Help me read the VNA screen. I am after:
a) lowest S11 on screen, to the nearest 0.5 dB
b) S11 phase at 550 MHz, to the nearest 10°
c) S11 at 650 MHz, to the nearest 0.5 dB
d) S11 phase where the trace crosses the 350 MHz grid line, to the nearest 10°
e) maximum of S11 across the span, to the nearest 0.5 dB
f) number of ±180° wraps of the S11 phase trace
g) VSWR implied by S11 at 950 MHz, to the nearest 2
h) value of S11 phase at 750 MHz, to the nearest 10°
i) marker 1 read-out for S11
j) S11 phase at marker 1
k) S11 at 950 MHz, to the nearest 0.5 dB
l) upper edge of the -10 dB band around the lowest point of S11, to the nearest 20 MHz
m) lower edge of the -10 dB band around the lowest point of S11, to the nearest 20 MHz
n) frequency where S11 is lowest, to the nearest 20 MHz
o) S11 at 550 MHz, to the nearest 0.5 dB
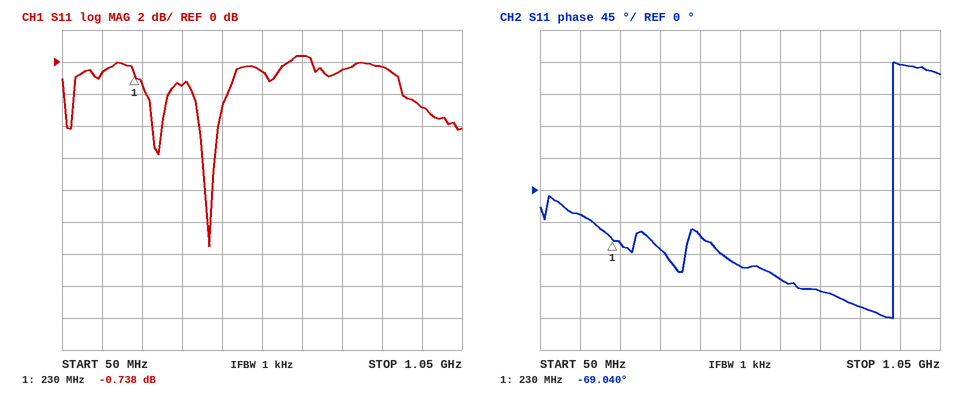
-11.5 dB
-110°
0.5 dB
-80°
0.5 dB
1
6
-140°
-0.738 dB
-69.040°
-3.0 dB
420 MHz
420 MHz
420 MHz
-0.5 dB
